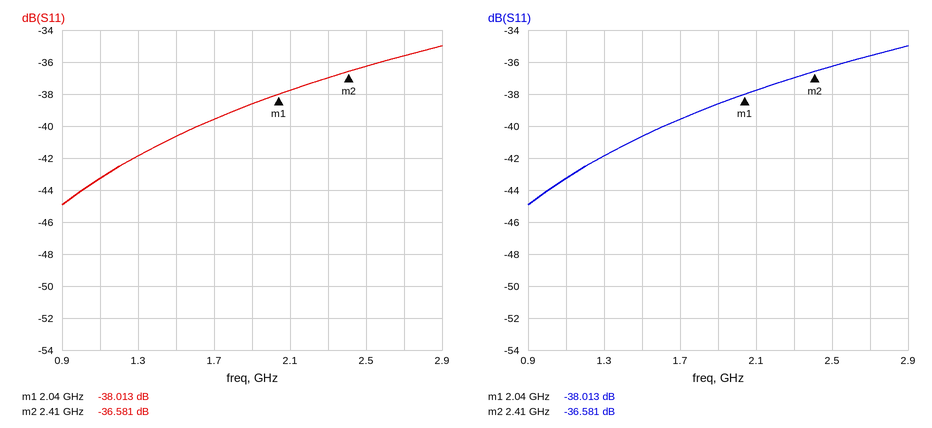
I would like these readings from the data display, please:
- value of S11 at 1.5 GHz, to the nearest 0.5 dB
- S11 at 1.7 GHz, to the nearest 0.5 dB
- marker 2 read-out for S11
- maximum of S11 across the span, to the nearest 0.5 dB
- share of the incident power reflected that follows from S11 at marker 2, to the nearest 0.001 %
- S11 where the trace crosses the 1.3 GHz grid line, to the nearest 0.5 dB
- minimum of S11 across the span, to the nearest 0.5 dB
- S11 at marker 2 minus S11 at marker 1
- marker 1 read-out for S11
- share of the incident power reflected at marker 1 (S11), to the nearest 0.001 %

-40.5 dB
-39.5 dB
-36.581 dB
-35.0 dB
0.022 %
-42.0 dB
-45.0 dB
1.432 dB
-38.013 dB
0.016 %
